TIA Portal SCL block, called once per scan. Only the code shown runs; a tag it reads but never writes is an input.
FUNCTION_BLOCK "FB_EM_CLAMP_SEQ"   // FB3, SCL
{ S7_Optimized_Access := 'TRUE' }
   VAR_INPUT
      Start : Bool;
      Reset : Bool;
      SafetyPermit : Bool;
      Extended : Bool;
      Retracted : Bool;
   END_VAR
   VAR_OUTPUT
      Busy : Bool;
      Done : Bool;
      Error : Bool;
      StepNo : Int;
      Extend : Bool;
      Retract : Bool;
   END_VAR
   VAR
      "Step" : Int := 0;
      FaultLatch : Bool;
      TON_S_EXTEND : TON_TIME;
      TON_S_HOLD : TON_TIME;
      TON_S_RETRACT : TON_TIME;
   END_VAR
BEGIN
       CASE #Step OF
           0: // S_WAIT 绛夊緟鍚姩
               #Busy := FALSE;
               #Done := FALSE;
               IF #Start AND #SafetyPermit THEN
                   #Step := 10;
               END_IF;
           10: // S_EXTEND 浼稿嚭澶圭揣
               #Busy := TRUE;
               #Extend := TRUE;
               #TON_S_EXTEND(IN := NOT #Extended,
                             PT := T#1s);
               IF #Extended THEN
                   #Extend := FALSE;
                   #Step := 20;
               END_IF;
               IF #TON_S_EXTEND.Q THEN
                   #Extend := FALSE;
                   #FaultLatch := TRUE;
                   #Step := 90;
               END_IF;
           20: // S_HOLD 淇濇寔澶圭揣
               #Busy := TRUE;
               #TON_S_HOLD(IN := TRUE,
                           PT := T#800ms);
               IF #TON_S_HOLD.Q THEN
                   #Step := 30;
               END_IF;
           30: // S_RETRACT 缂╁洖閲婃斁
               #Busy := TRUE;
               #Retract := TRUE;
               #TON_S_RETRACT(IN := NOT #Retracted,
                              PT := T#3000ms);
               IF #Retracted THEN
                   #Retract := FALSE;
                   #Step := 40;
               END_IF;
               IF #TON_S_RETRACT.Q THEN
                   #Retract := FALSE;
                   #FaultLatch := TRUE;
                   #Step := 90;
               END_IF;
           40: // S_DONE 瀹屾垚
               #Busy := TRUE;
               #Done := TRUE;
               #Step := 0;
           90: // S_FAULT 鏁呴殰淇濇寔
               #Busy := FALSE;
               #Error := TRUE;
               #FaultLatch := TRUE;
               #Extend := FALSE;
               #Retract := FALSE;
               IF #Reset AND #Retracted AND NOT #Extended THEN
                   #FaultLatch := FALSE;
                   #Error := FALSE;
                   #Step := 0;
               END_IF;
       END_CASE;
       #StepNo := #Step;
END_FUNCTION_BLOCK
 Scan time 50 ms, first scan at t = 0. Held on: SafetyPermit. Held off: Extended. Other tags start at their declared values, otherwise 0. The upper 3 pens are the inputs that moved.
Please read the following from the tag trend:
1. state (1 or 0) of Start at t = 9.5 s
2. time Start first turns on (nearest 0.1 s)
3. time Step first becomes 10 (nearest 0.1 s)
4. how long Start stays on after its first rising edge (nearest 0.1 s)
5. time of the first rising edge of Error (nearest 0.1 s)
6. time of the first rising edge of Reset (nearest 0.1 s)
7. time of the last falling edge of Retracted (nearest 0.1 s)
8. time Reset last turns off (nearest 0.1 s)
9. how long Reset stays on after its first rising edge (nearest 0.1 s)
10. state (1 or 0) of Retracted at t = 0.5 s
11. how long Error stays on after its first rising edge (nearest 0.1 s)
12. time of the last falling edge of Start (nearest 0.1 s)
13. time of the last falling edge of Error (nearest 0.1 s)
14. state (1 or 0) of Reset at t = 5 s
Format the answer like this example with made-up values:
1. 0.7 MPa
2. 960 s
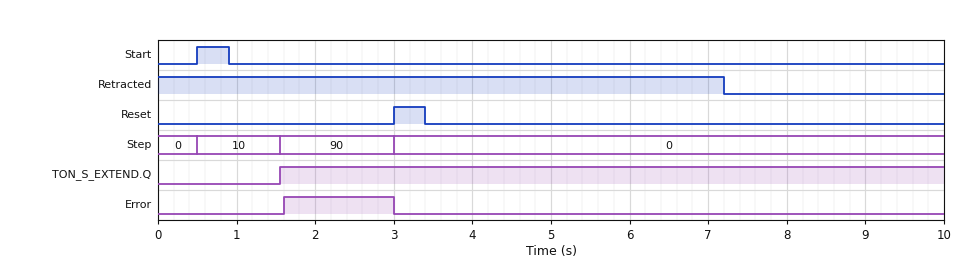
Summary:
1. 0
2. 0.5 s
3. 0.5 s
4. 0.4 s
5. 1.6 s
6. 3.0 s
7. 7.2 s
8. 3.4 s
9. 0.4 s
10. 1
11. 1.4 s
12. 0.9 s
13. 3.0 s
14. 0
